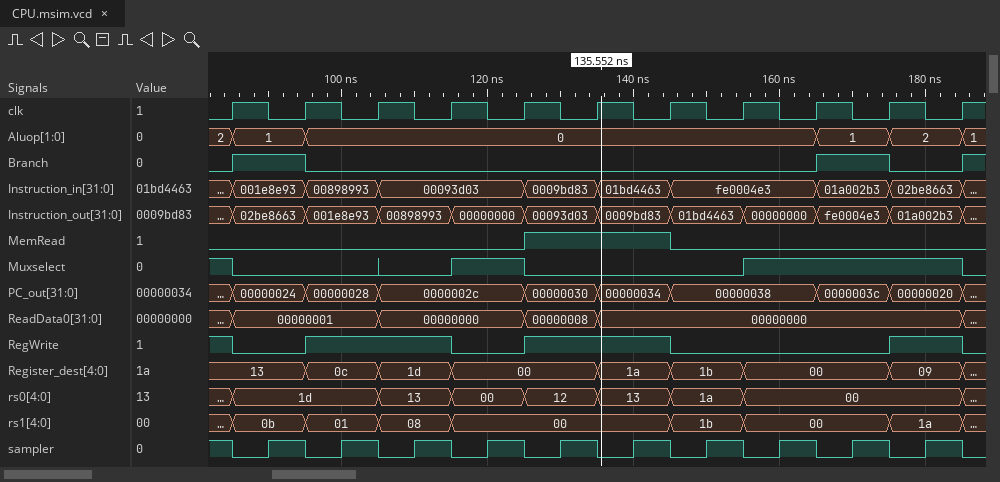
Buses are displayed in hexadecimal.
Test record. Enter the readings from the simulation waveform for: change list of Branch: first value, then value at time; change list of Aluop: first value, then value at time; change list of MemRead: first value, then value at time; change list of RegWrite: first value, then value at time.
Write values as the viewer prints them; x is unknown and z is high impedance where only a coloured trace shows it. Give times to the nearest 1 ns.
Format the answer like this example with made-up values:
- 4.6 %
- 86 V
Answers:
- 0, 1 at 85 ns, 0 at 95 ns, 1 at 165 ns, 0 at 175 ns, 1 at 185 ns
- 2, 1 at 85 ns, 0 at 95 ns, 1 at 165 ns, 2 at 175 ns, 1 at 185 ns
- 0, 1 at 125 ns, 0 at 145 ns
- 1, 0 at 85 ns, 1 at 95 ns, 0 at 115 ns, 1 at 125 ns, 0 at 145 ns, 1 at 175 ns, 0 at 185 ns
